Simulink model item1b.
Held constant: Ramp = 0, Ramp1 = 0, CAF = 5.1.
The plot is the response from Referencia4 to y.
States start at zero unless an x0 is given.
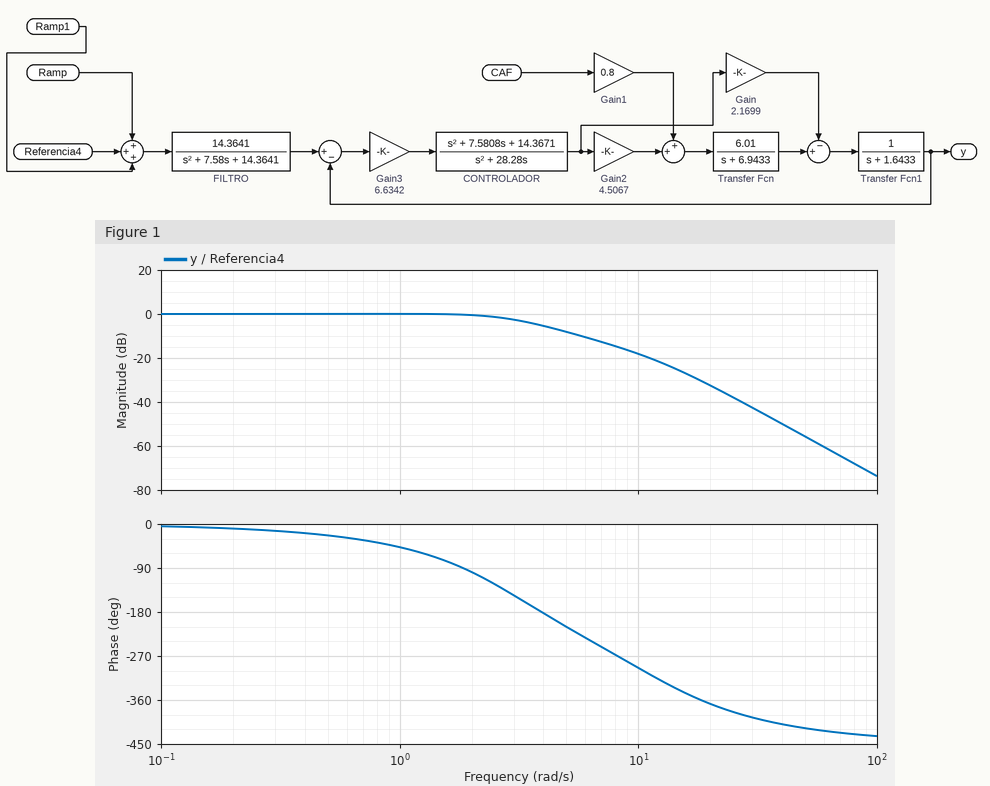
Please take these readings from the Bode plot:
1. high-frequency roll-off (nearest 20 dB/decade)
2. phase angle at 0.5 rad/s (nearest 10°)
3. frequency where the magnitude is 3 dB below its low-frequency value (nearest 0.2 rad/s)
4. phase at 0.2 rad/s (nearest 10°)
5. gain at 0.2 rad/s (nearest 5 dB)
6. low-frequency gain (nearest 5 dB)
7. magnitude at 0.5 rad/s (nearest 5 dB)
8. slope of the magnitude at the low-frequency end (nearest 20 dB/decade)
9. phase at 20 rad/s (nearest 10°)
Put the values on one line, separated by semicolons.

-60 dB/decade; -20°; 3.2 rad/s; -10°; 0 dB; 0 dB; 0 dB; 0 dB/decade; -370°
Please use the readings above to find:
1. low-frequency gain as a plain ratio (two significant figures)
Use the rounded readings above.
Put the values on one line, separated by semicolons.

1.0
